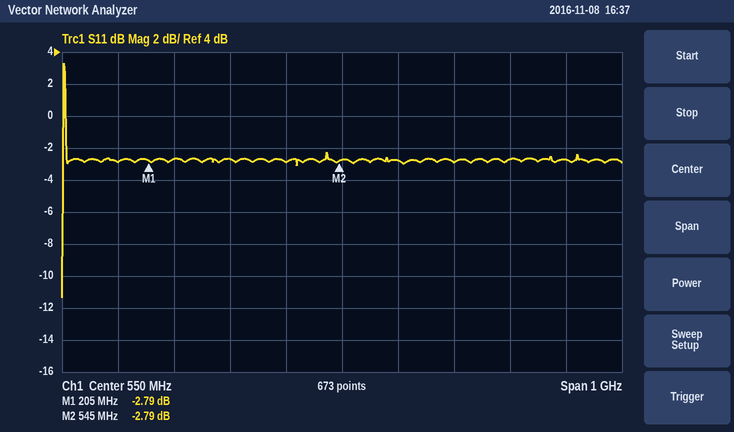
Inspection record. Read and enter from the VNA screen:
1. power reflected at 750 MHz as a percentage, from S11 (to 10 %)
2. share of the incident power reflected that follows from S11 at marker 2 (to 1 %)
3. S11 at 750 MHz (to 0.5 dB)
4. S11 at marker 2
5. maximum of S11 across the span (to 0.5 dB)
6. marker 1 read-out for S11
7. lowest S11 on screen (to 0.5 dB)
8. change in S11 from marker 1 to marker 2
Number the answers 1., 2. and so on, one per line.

1. 50 %
2. 53 %
3. -3.0 dB
4. -2.79 dB
5. 3.5 dB
6. -2.79 dB
7. -11.5 dB
8. 0.00 dB
